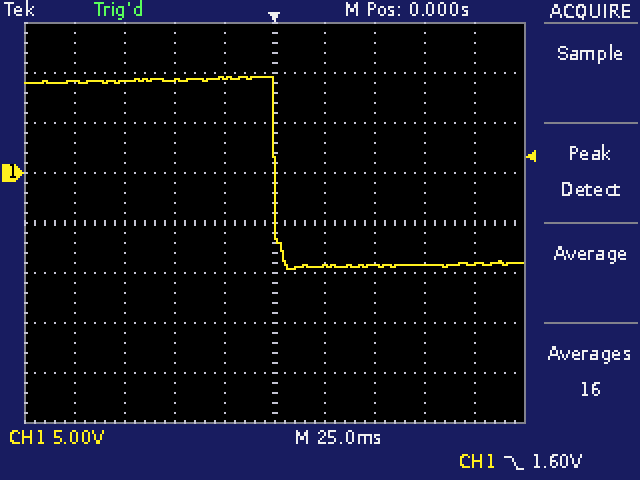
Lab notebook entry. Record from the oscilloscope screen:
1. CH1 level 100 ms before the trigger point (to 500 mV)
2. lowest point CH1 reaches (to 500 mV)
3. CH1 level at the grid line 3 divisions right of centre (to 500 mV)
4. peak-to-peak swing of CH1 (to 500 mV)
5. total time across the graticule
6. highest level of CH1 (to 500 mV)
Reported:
9.0 V
-9.5 V
-9.0 V
19.0 V
250 ms
9.5 V
